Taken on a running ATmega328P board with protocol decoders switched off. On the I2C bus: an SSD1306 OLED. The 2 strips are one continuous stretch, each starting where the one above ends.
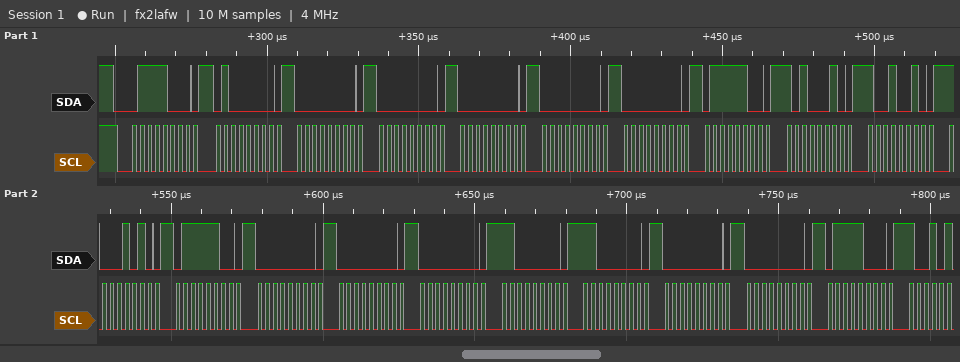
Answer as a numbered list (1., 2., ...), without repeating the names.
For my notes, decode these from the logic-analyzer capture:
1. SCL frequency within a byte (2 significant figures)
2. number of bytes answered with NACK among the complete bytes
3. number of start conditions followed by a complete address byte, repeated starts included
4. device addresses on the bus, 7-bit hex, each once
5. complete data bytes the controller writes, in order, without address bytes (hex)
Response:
1. 400 kHz
2. 0
3. 1
4. 0x3C
5. 40 00 00 00 00 00 7C A2 92 8A 7C 00 00 00 C0 C0 00 00 78
